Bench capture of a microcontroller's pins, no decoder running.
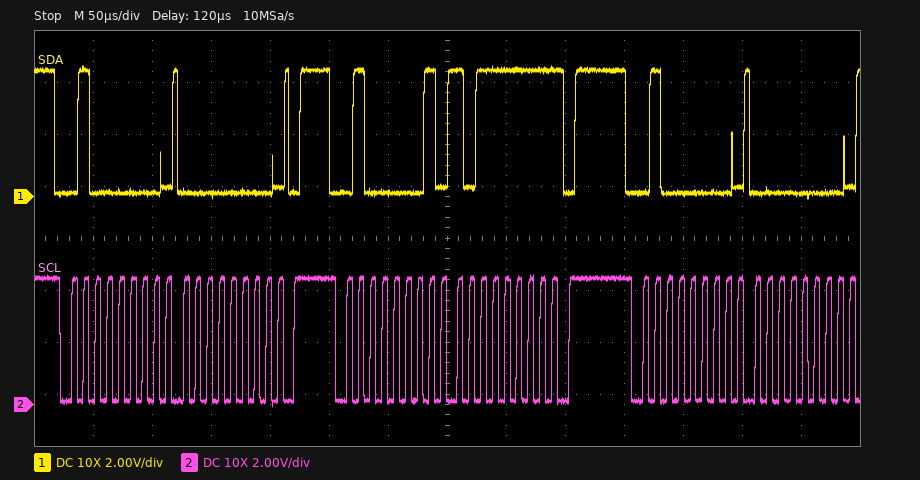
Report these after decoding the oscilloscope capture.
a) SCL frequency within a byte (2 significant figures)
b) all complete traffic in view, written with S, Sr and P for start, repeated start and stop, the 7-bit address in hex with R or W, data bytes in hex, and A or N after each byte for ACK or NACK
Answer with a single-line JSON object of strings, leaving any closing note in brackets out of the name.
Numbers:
{"SCL frequency within a byte": "100 kHz", "all complete traffic in view, written with S, Sr and P for start, repeated start and stop, the 7-bit address in hex with R or W, data bytes in hex, and A or N after each byte for ACK or NACK": "S 20W A 00 A P S 20R A BF N P S 20W A 00 A"}
